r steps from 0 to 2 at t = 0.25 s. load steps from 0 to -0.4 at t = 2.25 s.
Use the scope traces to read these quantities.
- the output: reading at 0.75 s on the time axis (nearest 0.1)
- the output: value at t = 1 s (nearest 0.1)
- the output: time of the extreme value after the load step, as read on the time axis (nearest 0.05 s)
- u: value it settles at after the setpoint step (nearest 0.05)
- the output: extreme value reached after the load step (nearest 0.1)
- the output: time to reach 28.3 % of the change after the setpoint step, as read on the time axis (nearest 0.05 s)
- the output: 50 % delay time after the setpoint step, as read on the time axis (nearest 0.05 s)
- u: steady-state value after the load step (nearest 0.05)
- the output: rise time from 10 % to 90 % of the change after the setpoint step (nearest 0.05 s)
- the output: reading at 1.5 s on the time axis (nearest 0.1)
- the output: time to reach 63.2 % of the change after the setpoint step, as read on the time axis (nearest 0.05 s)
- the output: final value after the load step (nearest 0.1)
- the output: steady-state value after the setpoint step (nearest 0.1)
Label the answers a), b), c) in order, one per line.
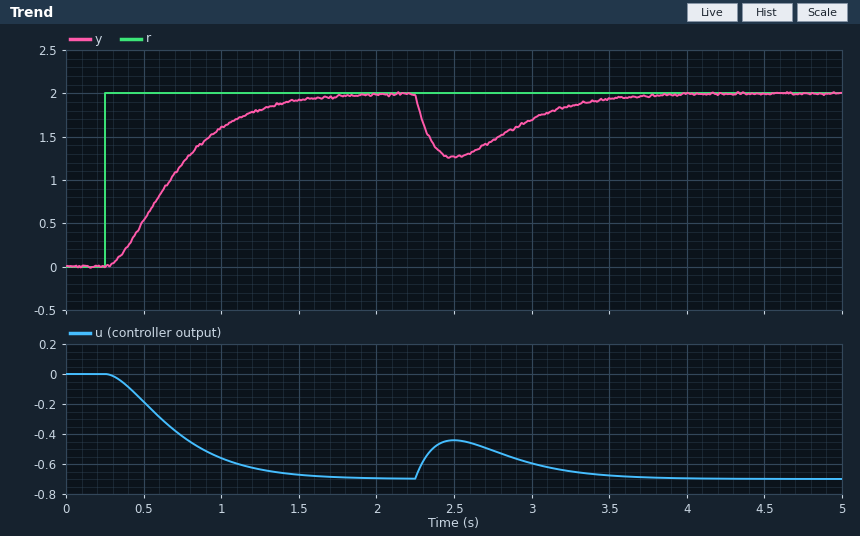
a) 1.2
b) 1.6
c) 2.50 s
d) -0.70
e) 1.3
f) 0.50 s
g) 0.65 s
h) -0.70
i) 0.85 s
j) 1.9
k) 0.80 s
l) 2.0
m) 2.0
